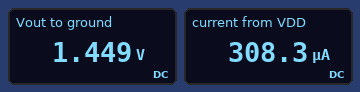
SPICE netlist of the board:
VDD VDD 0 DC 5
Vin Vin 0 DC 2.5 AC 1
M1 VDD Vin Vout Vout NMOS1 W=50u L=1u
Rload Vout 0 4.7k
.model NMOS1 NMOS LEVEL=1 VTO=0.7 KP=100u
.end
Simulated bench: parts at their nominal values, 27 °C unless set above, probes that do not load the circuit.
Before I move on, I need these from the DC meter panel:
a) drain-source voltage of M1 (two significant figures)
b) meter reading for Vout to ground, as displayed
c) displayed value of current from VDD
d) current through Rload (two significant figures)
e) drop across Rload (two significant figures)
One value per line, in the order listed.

3.6 V
1.449 V
308.3 µA
310 µA
1.4 V
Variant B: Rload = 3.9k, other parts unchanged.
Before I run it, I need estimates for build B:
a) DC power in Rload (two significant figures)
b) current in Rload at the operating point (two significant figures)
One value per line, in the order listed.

520 µW
360 µA
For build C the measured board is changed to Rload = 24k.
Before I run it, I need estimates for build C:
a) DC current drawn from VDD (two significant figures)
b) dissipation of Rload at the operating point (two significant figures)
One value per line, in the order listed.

68 µA
110 µW
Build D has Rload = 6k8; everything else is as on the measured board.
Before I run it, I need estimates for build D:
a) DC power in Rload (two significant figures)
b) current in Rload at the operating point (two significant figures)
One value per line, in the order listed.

330 µW
220 µA
